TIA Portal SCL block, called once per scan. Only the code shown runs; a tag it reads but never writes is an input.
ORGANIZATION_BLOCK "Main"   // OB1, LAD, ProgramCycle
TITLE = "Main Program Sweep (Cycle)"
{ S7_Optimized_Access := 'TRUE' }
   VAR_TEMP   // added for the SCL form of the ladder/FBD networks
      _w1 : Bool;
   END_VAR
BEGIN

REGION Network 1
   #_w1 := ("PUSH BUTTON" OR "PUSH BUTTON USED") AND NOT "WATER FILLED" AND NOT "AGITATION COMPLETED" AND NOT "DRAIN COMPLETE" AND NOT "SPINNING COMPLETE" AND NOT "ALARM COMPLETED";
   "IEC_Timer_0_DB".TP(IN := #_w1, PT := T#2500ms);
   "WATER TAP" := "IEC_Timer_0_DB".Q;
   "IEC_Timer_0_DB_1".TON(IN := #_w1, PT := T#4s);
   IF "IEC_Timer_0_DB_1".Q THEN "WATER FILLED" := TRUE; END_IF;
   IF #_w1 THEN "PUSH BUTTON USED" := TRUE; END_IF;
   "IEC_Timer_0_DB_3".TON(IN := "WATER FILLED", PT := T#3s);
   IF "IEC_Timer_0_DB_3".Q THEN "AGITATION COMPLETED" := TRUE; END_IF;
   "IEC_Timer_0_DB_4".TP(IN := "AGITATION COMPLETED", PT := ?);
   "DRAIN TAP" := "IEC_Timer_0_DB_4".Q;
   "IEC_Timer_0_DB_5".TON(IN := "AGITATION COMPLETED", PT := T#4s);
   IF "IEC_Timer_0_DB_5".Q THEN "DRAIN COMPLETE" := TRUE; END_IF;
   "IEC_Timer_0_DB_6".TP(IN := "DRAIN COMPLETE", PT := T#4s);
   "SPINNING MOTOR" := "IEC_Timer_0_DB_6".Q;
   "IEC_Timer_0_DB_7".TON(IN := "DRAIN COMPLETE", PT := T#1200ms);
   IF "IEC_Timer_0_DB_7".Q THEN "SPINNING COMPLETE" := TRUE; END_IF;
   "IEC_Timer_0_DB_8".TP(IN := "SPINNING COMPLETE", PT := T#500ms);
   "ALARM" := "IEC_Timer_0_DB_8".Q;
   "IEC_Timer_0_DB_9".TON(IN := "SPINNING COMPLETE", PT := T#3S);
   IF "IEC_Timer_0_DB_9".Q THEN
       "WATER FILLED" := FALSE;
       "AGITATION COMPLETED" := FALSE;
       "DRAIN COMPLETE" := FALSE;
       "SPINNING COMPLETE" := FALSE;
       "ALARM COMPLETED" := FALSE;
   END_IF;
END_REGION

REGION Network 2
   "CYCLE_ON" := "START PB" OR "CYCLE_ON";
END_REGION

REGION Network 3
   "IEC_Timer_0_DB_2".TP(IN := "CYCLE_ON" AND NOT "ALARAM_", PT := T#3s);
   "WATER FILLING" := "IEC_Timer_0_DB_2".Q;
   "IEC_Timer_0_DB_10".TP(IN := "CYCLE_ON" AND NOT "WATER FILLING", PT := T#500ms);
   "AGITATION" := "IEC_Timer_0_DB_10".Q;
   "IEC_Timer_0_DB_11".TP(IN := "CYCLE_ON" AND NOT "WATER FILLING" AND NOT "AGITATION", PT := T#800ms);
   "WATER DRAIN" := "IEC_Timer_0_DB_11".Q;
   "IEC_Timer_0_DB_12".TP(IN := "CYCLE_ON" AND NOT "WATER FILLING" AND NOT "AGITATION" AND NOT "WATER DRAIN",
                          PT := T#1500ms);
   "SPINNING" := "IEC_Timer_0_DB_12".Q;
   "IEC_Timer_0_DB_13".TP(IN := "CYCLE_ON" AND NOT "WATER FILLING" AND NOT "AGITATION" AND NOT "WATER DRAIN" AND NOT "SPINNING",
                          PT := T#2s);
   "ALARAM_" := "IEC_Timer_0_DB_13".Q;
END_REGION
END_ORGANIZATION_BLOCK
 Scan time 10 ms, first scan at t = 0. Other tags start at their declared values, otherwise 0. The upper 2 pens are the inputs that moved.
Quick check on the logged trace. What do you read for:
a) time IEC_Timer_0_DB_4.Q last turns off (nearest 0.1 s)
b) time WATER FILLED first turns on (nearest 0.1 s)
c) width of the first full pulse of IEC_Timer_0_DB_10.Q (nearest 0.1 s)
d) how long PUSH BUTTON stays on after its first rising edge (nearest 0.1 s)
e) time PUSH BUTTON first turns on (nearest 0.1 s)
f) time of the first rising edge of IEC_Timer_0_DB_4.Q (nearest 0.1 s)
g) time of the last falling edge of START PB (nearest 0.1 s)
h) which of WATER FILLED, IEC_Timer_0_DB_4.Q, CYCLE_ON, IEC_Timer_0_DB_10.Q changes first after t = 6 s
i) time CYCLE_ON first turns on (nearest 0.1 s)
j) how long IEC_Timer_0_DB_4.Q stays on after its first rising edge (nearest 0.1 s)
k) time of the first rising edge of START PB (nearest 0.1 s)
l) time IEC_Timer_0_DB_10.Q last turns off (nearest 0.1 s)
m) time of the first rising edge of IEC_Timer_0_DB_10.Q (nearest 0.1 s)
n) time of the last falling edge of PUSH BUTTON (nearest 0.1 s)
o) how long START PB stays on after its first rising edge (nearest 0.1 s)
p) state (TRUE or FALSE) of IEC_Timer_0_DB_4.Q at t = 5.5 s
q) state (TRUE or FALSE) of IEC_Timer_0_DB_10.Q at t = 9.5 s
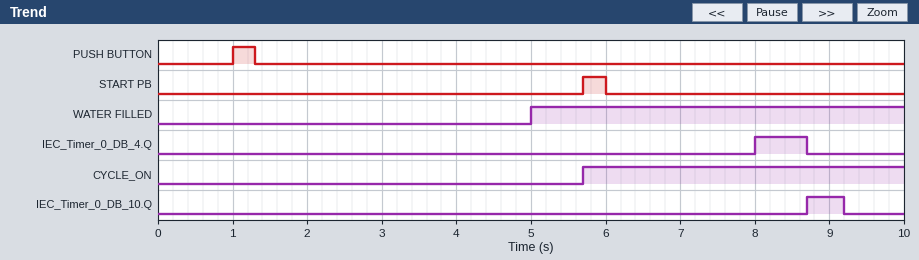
8.7 s
5.0 s
0.5 s
0.3 s
1.0 s
8.0 s
6.0 s
IEC_Timer_0_DB_4.Q
5.7 s
0.7 s
5.7 s
9.2 s
8.7 s
1.3 s
0.3 s
FALSE
FALSE
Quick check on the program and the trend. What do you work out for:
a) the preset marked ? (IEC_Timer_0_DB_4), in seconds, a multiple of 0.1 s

0.7 s
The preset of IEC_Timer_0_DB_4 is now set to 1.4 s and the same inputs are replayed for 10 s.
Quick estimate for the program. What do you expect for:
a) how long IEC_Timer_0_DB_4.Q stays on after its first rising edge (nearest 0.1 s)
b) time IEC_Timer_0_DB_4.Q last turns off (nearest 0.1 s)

1.4 s
9.4 s
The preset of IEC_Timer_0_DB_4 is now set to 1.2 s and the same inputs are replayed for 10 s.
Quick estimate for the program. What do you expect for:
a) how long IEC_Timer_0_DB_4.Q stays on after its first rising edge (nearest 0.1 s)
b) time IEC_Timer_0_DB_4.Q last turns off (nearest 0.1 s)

1.2 s
9.2 s
